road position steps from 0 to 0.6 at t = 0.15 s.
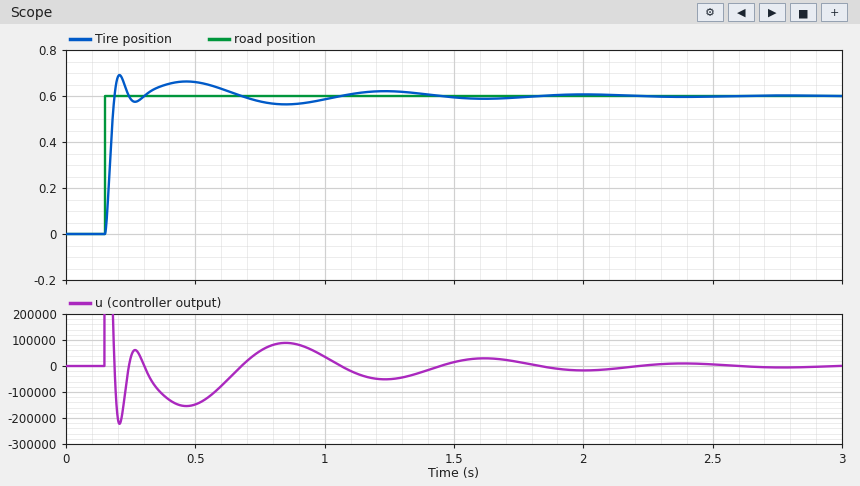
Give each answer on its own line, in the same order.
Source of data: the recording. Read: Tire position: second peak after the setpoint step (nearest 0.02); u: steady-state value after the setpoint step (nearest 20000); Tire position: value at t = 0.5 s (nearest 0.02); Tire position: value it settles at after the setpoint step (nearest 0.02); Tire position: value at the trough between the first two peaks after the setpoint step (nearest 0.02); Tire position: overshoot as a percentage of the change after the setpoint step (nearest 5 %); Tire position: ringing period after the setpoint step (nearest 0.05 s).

0.66
0
0.66
0.60
0.58
15 %
0.25 s
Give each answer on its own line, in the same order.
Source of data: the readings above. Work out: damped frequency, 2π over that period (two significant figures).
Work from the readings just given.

25 rad/s
